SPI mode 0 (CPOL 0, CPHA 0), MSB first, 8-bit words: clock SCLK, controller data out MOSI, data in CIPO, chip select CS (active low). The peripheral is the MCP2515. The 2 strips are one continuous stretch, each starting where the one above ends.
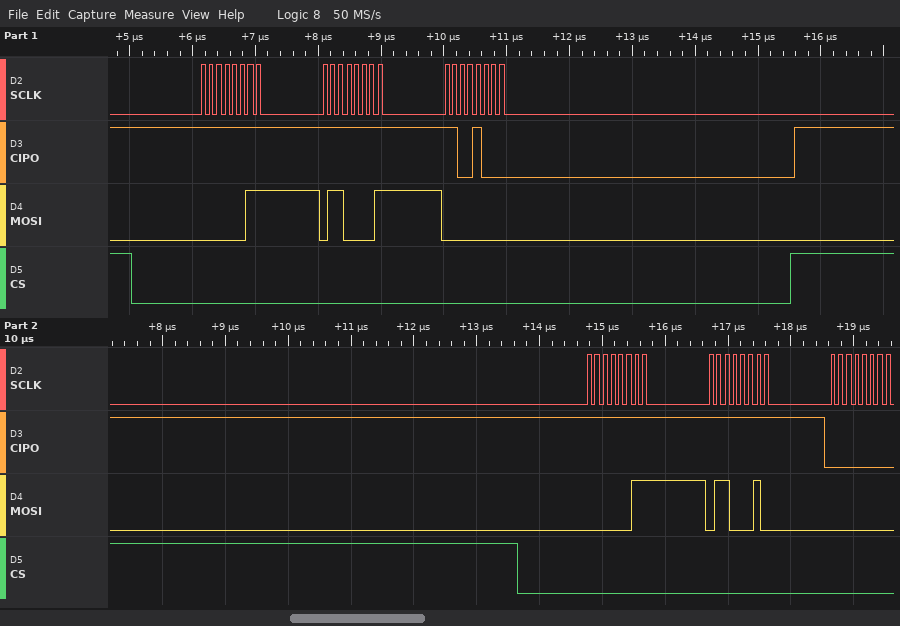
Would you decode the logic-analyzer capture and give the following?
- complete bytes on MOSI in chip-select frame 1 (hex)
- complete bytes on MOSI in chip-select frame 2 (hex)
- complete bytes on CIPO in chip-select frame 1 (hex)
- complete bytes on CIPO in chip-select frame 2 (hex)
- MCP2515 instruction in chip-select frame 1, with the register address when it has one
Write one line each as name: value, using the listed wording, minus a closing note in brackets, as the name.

complete bytes on MOSI in chip-select frame 1: 0x03 0x61 0x00
complete bytes on MOSI in chip-select frame 2: 0x03 0x62 0x00
complete bytes on CIPO in chip-select frame 1: 0xFF 0xFF 0xC8
complete bytes on CIPO in chip-select frame 2: 0xFF 0xFF 0x00
MCP2515 instruction in chip-select frame 1, with the register address when it has one: READ 0x61
